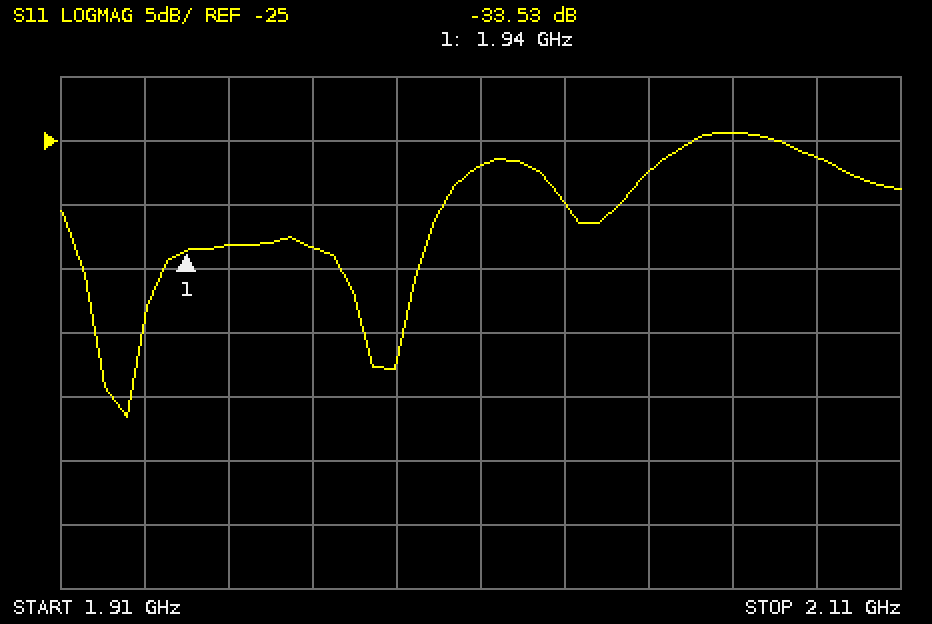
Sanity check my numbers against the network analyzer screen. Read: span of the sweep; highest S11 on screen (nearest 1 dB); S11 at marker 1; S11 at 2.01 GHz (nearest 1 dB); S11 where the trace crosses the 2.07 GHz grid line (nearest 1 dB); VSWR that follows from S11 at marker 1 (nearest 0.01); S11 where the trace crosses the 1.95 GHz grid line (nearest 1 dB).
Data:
200 MHz
-24 dB
-33.53 dB
-27 dB
-24 dB
1.04
-33 dB
